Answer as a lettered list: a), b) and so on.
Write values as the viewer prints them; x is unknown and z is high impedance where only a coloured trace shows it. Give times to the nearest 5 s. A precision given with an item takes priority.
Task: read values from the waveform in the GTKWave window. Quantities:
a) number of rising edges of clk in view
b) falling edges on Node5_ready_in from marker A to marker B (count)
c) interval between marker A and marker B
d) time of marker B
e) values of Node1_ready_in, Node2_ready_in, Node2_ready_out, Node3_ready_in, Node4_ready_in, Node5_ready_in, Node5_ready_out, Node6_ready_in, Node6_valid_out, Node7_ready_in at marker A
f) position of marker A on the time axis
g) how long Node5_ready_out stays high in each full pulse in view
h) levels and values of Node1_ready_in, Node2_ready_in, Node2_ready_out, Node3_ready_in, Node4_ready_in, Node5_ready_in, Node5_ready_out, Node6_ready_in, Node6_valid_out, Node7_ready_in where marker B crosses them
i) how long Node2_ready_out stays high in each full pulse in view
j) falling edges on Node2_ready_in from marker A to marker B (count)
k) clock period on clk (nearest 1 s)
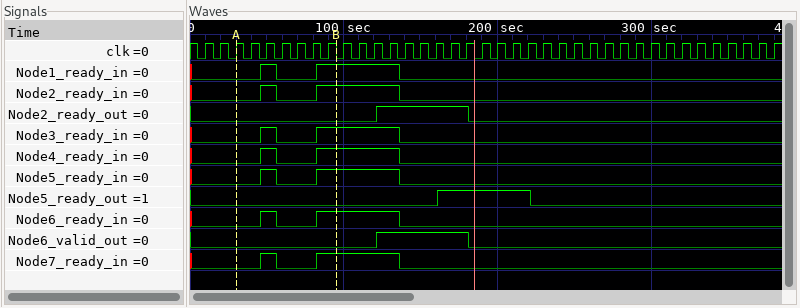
a) 38
b) 1
c) 65 s
d) 95 s
e) Node1_ready_in=0, Node2_ready_in=0, Node2_ready_out=0, Node3_ready_in=0, Node4_ready_in=0, Node5_ready_in=0, Node5_ready_out=0, Node6_ready_in=0, Node6_valid_out=0, Node7_ready_in=0
f) 30 s
g) 60 s
h) Node1_ready_in=1, Node2_ready_in=1, Node2_ready_out=0, Node3_ready_in=1, Node4_ready_in=1, Node5_ready_in=1, Node5_ready_out=0, Node6_ready_in=1, Node6_valid_out=0, Node7_ready_in=1
i) 60 s
j) 1
k) 10 s
